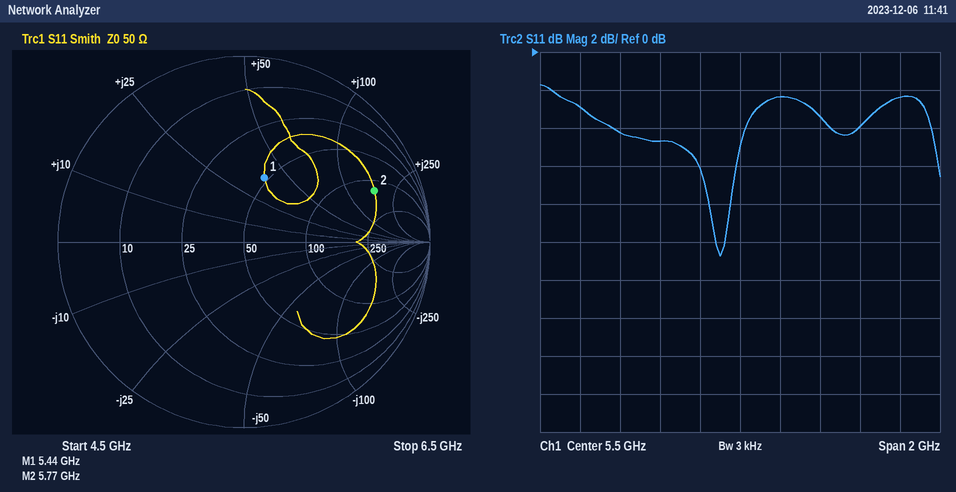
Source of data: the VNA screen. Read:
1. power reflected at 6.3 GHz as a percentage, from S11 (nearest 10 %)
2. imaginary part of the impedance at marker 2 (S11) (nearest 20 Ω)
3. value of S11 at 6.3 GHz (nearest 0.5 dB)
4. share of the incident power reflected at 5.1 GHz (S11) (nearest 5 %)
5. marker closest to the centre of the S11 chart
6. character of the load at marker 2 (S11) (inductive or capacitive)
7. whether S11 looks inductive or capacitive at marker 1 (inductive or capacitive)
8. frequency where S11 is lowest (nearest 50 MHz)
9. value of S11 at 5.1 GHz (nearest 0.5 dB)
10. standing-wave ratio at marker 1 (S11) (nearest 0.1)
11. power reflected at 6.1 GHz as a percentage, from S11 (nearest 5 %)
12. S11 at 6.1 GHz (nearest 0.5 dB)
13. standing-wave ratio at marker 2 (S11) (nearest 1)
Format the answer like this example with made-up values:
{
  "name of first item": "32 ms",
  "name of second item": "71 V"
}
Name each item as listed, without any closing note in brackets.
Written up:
{
  "power reflected at 6.3 GHz as a percentage, from S11": "60 %",
  "imaginary part of the impedance at marker 2 (S11)": "+160 Ω",
  "value of S11 at 6.3 GHz": "-2.5 dB",
  "share of the incident power reflected at 5.1 GHz (S11)": "35 %",
  "marker closest to the centre of the S11 chart": "marker 1",
  "character of the load at marker 2 (S11)": "inductive",
  "whether S11 looks inductive or capacitive at marker 1": "inductive",
  "frequency where S11 is lowest": "5.40 GHz",
  "value of S11 at 5.1 GHz": "-4.5 dB",
  "standing-wave ratio at marker 1 (S11)": "2.1",
  "power reflected at 6.1 GHz as a percentage, from S11": "40 %",
  "S11 at 6.1 GHz": "-4.0 dB",
  "standing-wave ratio at marker 2 (S11)": "7"
}
